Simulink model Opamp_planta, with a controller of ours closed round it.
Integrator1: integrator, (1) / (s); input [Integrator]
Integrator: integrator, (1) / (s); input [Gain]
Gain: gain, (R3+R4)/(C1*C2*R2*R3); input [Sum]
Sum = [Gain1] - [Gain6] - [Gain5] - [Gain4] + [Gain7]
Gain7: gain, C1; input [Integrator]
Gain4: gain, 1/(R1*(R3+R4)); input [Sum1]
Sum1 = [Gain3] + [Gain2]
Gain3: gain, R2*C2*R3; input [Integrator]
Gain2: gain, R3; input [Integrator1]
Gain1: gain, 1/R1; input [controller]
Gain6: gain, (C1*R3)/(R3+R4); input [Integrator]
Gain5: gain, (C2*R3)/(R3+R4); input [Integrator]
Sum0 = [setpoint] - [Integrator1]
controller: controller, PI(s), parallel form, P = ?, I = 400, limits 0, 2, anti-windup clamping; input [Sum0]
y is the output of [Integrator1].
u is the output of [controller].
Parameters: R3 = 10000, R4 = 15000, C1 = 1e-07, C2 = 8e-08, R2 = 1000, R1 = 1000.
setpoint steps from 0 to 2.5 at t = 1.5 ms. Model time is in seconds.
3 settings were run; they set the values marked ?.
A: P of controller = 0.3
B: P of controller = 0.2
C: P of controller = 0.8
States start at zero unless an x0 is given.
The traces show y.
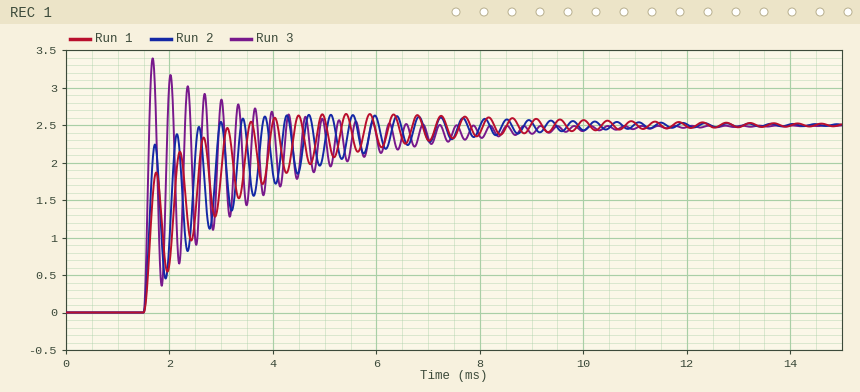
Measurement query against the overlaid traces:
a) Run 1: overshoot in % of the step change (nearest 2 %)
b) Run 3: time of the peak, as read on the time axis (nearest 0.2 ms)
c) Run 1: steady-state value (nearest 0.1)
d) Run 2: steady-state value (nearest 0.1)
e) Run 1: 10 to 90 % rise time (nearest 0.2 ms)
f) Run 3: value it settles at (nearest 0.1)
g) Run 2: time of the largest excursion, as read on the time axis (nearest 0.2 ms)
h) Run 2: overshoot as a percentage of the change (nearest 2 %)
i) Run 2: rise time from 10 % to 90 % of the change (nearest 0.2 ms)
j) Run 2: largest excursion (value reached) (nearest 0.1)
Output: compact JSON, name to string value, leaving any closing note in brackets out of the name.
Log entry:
{"Run 1: overshoot in % of the step change": "6 %", "Run 3: time of the peak, as read on the time axis": "1.6 ms", "Run 1: steady-state value": "2.5", "Run 2: steady-state value": "2.5", "Run 1: 10 to 90 % rise time": "1.0 ms", "Run 3: value it settles at": "2.5", "Run 2: time of the largest excursion, as read on the time axis": "5.2 ms", "Run 2: overshoot as a percentage of the change": "6 %", "Run 2: rise time from 10 % to 90 % of the change": "0.6 ms", "Run 2: largest excursion (value reached)": "2.6"}
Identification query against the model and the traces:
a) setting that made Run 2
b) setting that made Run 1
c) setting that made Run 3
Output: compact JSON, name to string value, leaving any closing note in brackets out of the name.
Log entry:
{"setting that made Run 2": "A", "setting that made Run 1": "B", "setting that made Run 3": "C"}
